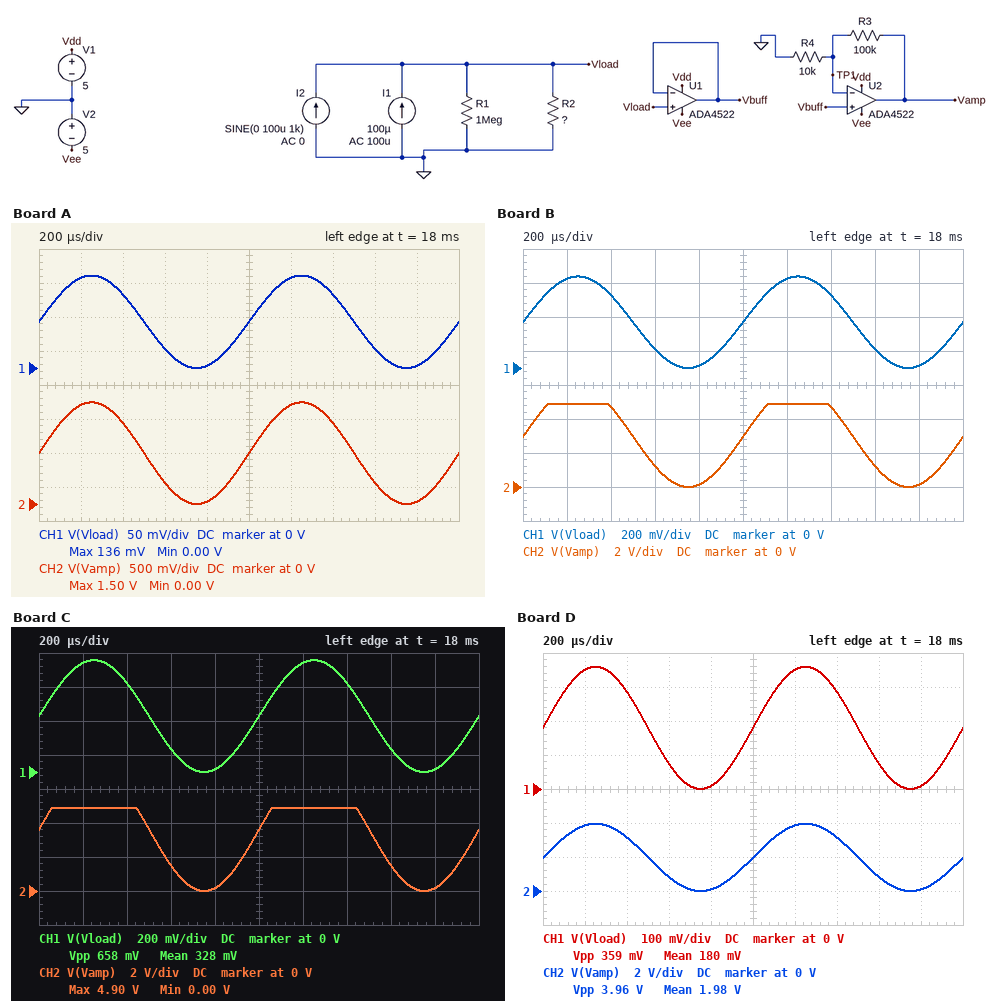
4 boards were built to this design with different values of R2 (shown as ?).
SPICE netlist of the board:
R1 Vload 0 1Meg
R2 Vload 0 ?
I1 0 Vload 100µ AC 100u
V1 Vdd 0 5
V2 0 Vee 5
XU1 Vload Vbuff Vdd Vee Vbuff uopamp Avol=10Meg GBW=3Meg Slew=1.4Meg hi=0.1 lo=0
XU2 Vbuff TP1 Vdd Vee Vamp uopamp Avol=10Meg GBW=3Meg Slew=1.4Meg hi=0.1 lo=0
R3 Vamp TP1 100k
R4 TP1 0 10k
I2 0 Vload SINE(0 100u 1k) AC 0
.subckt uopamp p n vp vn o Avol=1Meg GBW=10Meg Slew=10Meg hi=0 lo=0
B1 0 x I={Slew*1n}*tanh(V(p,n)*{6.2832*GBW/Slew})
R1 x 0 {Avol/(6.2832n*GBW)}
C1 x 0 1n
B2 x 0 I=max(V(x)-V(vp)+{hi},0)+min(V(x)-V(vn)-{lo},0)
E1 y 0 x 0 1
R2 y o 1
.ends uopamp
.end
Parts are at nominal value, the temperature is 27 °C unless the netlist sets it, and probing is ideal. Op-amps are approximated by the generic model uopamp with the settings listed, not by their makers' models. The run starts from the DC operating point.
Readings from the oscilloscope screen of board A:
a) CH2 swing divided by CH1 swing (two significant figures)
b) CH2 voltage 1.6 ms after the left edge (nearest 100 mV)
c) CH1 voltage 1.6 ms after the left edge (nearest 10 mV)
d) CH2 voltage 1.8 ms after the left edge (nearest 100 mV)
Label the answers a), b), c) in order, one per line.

a) 11
b) 300 mV
c) 30 mV
d) 0 V
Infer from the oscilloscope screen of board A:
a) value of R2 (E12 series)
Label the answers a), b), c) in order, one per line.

a) 680 Ω
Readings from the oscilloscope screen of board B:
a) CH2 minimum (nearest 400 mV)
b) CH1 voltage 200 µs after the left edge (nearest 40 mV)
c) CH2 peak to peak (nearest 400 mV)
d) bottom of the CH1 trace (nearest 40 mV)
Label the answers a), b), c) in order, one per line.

a) 0 V
b) 520 mV
c) 4.8 V
d) 0 V
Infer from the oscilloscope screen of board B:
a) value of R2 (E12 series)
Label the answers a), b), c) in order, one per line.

a) 2.7 kΩ
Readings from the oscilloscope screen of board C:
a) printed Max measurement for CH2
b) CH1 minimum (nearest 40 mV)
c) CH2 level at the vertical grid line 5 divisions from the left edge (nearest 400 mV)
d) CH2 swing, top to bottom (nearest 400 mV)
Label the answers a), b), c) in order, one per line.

a) 4.90 V
b) 0 V
c) 3.6 V
d) 4.8 V
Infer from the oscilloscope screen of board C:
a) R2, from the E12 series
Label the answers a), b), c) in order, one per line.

a) 3.3 kΩ
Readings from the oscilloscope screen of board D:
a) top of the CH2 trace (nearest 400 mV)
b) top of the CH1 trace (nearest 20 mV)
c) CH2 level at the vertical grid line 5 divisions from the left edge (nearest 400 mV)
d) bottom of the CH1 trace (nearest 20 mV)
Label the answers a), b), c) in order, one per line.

a) 4.0 V
b) 360 mV
c) 2.0 V
d) 0 V
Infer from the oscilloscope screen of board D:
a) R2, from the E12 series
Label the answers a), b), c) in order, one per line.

a) 1.8 kΩ
